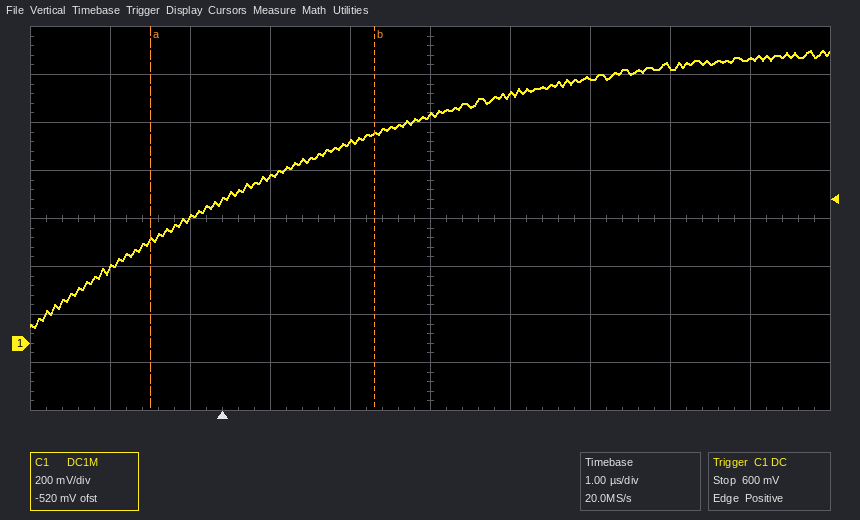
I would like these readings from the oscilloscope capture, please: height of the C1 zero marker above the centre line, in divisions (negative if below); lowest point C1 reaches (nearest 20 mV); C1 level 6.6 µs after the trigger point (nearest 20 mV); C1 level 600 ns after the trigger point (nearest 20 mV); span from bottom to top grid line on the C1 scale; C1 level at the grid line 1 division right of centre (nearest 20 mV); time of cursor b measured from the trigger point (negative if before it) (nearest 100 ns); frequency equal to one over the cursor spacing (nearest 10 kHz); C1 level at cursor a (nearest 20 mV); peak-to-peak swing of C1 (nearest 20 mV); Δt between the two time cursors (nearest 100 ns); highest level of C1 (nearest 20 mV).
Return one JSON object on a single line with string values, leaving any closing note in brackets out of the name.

{"height of the C1 zero marker above the centre line, in divisions": "-2.6 div", "lowest point C1 reaches": "60 mV", "C1 level 6.6 µs after the trigger point": "1.18 V", "C1 level 600 ns after the trigger point": "700 mV", "span from bottom to top grid line on the C1 scale": "1.6 V", "C1 level at the grid line 1 division right of centre": "1.04 V", "time of cursor b measured from the trigger point (negative if before it)": "+1.9 µs", "frequency equal to one over the cursor spacing": "360 kHz", "C1 level at cursor a": "420 mV", "peak-to-peak swing of C1": "1.16 V", "Δt between the two time cursors": "2.8 µs", "highest level of C1": "1.22 V"}
